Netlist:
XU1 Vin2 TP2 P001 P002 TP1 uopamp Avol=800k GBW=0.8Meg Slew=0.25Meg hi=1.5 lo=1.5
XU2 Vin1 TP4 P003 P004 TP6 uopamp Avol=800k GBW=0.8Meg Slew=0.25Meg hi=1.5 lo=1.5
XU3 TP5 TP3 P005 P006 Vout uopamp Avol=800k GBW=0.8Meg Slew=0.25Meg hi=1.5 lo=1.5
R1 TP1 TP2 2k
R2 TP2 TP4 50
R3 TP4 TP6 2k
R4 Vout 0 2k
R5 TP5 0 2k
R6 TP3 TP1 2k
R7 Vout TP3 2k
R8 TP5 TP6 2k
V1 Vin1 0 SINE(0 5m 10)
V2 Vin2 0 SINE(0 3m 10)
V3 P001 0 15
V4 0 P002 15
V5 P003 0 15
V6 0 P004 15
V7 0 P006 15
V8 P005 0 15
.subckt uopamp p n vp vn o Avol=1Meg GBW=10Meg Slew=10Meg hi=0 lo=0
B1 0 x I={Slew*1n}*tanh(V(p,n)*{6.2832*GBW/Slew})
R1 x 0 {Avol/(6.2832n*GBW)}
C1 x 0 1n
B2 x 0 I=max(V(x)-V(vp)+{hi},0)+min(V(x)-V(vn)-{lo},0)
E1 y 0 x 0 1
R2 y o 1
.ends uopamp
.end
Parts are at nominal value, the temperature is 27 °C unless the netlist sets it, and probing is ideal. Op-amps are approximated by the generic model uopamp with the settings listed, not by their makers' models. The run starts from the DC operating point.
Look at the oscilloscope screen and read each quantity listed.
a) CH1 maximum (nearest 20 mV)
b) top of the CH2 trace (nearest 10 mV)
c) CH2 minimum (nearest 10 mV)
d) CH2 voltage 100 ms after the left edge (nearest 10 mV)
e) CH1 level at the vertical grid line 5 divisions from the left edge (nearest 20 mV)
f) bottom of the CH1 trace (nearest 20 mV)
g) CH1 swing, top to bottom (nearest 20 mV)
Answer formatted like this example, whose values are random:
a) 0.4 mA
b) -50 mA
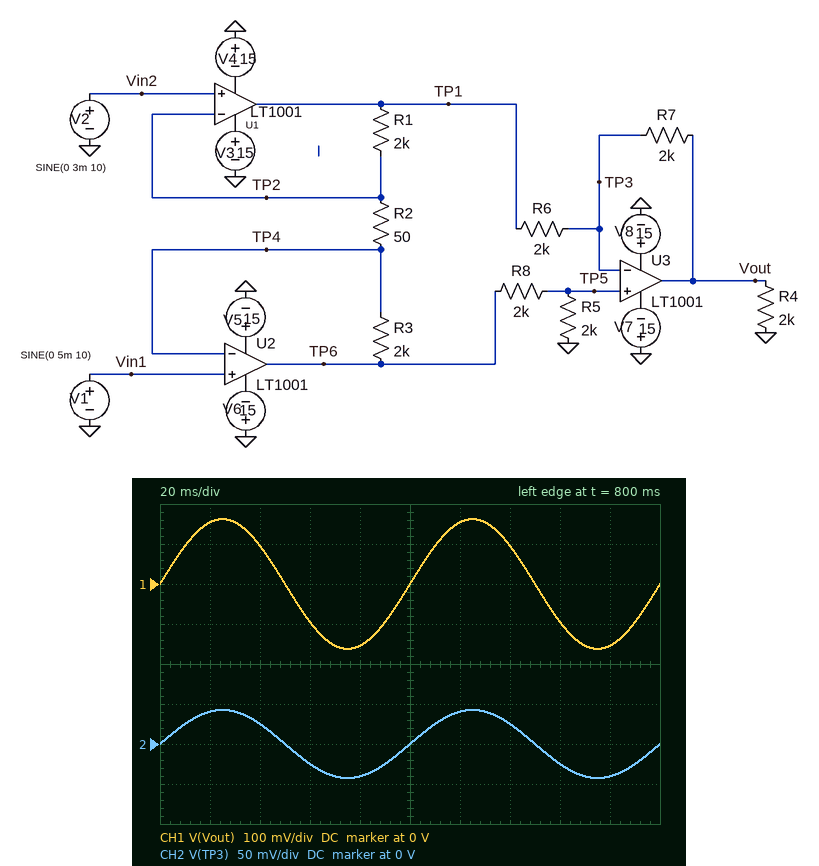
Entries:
a) 160 mV
b) 40 mV
c) -40 mV
d) 0 V
e) 0 V
f) -160 mV
g) 320 mV
